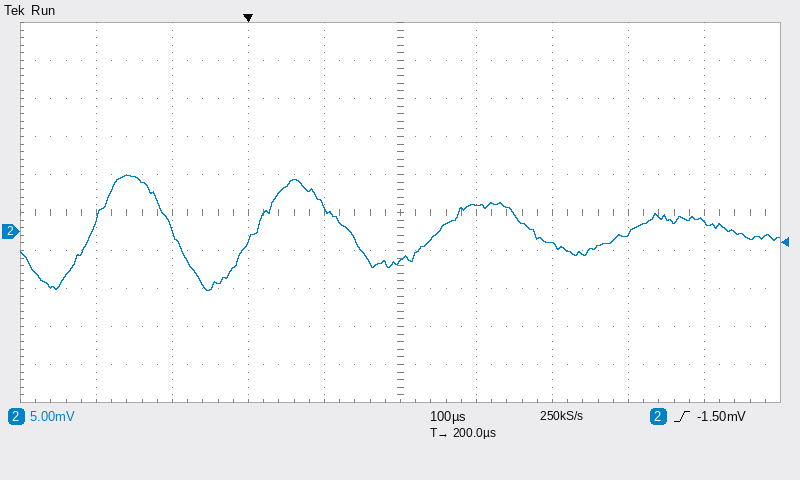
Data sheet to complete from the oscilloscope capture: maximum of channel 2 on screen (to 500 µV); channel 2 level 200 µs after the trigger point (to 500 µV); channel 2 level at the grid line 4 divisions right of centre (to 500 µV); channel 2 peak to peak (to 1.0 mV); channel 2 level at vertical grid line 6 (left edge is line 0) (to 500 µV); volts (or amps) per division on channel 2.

7.5 mV
-4.0 mV
1.5 mV
15.0 mV
3.5 mV
5 mV
